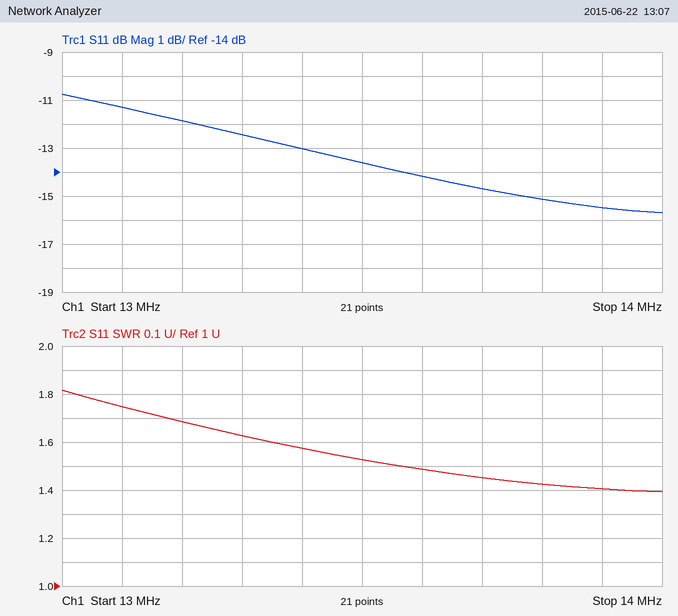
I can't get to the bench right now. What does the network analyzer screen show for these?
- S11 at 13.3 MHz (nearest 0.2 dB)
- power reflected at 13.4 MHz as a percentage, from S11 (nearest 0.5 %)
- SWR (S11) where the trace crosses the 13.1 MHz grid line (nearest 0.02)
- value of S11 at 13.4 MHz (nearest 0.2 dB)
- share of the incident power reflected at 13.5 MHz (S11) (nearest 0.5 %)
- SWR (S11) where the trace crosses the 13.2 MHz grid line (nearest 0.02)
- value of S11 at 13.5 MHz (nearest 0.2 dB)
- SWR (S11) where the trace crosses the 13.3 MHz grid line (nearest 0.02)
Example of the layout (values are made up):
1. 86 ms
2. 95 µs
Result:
1. -12.4 dB
2. 5.0 %
3. 1.74
4. -13.0 dB
5. 4.5 %
6. 1.68
7. -13.6 dB
8. 1.62
